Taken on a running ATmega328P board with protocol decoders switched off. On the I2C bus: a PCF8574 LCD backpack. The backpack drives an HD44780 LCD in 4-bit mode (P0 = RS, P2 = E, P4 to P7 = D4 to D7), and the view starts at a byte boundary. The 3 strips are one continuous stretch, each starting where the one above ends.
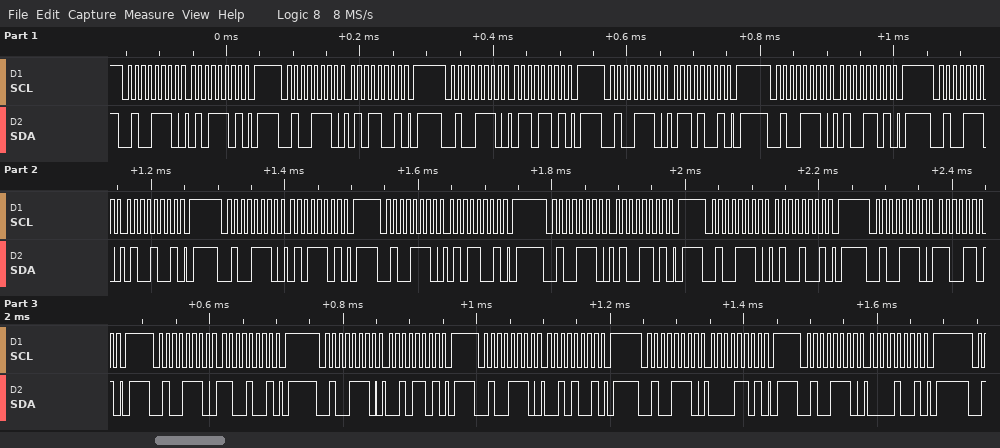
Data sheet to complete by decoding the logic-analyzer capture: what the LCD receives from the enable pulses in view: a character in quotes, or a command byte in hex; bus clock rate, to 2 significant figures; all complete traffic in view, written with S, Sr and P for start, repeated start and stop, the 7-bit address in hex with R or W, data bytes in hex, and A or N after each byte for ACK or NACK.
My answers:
'V' 'E' 'L' ' '
100 kHz
S 27W A 5D A P S 27W A 59 A P S 27W A 6D A P S 27W A 69 A P S 27W A 4D A P S 27W A 49 A P S 27W A 5D A P S 27W A 59 A P S 27W A 4D A P S 27W A 49 A P S 27W A CD A P S 27W A C9 A P S 27W A 2D A P S 27W A 29 A P S 27W A 0D A P S 27W A 09 A P
